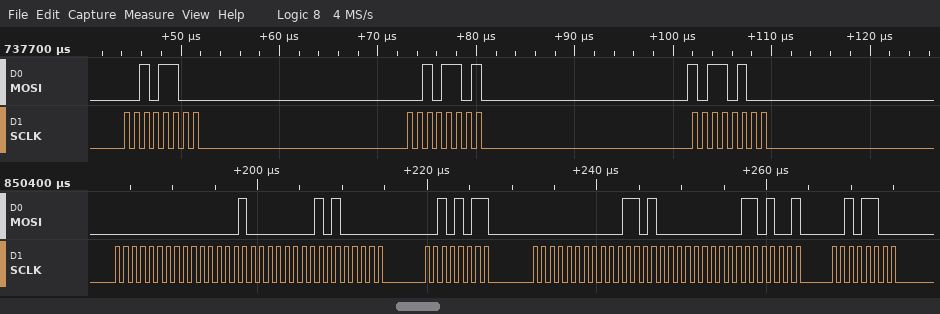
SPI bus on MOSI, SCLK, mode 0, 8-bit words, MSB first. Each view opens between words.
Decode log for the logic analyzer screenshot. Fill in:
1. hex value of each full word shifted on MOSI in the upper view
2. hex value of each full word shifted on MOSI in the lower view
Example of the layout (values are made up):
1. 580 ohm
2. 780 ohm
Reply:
1. 2C, 2D, B4
2. 00, 01, 00, A0, 2B, 00, 1A, 00, 69, 2C
